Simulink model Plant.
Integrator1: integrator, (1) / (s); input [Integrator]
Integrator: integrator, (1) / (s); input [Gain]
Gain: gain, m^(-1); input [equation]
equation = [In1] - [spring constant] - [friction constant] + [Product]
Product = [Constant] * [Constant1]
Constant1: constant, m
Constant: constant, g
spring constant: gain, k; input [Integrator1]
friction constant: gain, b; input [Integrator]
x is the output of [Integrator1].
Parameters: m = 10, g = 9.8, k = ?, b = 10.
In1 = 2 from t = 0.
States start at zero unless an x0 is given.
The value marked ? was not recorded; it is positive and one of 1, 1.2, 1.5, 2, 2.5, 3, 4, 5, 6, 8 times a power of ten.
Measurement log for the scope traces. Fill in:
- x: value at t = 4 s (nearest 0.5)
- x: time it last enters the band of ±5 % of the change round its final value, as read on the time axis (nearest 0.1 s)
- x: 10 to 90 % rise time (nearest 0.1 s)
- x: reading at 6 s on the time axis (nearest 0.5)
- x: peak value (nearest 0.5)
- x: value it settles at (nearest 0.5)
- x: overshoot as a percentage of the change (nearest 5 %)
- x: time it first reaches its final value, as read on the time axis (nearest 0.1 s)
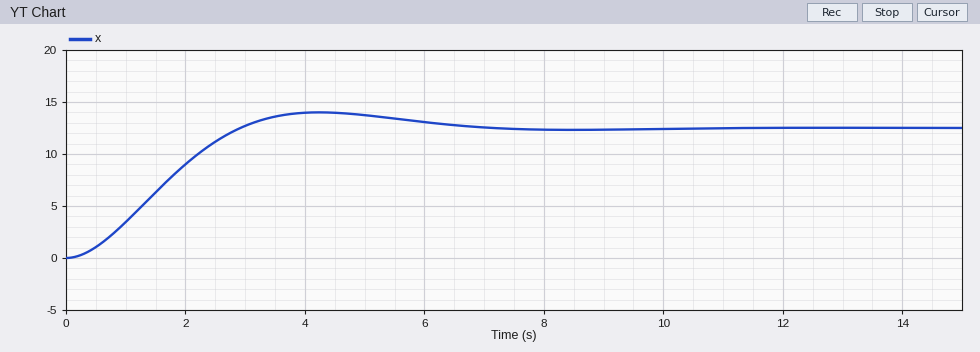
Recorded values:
14.0
5.9 s
2.0 s
13.0
14.0
12.5
10 %
2.9 s
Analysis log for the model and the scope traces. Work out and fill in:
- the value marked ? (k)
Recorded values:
8
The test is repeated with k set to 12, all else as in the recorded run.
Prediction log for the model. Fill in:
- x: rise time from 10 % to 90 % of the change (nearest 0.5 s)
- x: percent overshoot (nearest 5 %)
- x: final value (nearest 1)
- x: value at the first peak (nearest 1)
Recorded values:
1.5 s
20 %
8
10
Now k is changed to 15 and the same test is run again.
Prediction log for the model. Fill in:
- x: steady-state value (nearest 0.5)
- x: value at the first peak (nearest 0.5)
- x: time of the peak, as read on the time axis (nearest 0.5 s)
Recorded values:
6.5
8.5
3.0 s
